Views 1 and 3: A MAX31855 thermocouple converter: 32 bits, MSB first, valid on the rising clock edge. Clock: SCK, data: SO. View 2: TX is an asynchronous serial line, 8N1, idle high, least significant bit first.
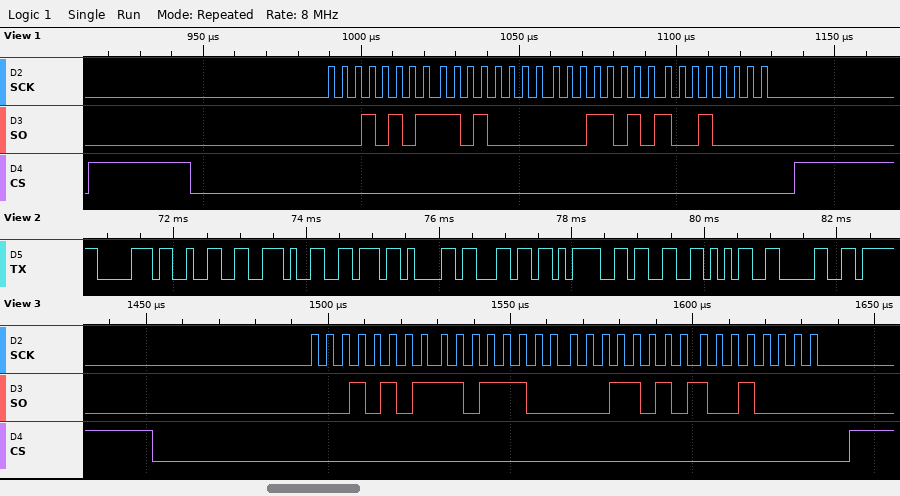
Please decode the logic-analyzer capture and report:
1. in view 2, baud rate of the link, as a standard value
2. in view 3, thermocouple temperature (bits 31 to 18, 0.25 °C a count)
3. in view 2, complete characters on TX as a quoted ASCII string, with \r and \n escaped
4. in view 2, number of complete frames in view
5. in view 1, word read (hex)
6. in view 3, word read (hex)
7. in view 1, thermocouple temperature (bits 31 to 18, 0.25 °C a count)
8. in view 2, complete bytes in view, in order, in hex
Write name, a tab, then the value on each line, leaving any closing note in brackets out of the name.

in view 2, baud rate of the link, as a standard value	9600 baud
in view 3, thermocouple temperature	349.75 °C
in view 2, complete characters on TX as a quoted ASCII string, with \r and \n escaped	"p2.val=350"
in view 2, number of complete frames in view	10
in view 1, word read	0x15D01A90
in view 3, word read	0x15DC1A90
in view 1, thermocouple temperature	349.00 °C
in view 2, complete bytes in view, in order, in hex	0x70 0x32 0x2E 0x76 0x61 0x6C 0x3D 0x33 0x35 0x30
